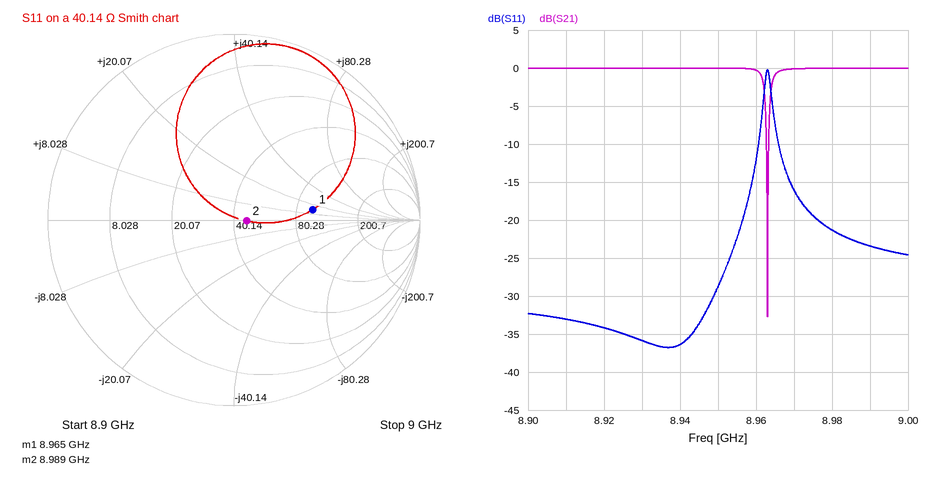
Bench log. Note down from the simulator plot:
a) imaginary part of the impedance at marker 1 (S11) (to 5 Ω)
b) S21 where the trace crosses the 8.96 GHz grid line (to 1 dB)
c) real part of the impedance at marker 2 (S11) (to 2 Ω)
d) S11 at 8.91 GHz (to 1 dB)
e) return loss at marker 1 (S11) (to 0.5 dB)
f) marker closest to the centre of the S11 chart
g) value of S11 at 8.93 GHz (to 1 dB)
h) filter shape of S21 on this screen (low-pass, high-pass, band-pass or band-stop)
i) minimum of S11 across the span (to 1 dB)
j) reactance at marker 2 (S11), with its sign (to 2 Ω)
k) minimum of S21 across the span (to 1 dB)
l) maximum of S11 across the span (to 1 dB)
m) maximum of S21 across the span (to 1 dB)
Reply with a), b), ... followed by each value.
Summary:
a) +15 Ω
b) 0 dB
c) 46 Ω
d) -33 dB
e) 7.5 dB
f) marker 2
g) -36 dB
h) band-stop
i) -37 dB
j) 0 Ω
k) -33 dB
l) 0 dB
m) 0 dB
